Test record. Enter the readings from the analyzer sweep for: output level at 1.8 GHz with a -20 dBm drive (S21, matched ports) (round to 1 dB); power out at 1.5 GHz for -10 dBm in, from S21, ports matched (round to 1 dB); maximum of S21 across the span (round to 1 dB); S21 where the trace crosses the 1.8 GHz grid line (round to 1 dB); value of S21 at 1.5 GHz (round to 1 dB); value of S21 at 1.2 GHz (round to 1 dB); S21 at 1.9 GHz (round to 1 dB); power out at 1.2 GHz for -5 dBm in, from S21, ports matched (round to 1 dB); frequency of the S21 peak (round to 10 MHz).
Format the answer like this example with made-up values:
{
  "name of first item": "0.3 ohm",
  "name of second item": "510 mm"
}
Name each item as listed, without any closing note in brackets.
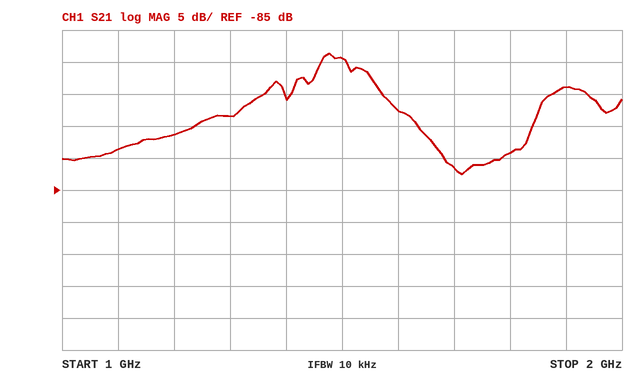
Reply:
{
  "output level at 1.8 GHz with a -20 dBm drive (S21, matched ports)": "-99 dBm",
  "power out at 1.5 GHz for -10 dBm in, from S21, ports matched": "-74 dBm",
  "maximum of S21 across the span": "-64 dB",
  "S21 where the trace crosses the 1.8 GHz grid line": "-79 dB",
  "value of S21 at 1.5 GHz": "-64 dB",
  "value of S21 at 1.2 GHz": "-76 dB",
  "S21 at 1.9 GHz": "-69 dB",
  "power out at 1.2 GHz for -5 dBm in, from S21, ports matched": "-81 dBm",
  "frequency of the S21 peak": "1.48 GHz"
}
